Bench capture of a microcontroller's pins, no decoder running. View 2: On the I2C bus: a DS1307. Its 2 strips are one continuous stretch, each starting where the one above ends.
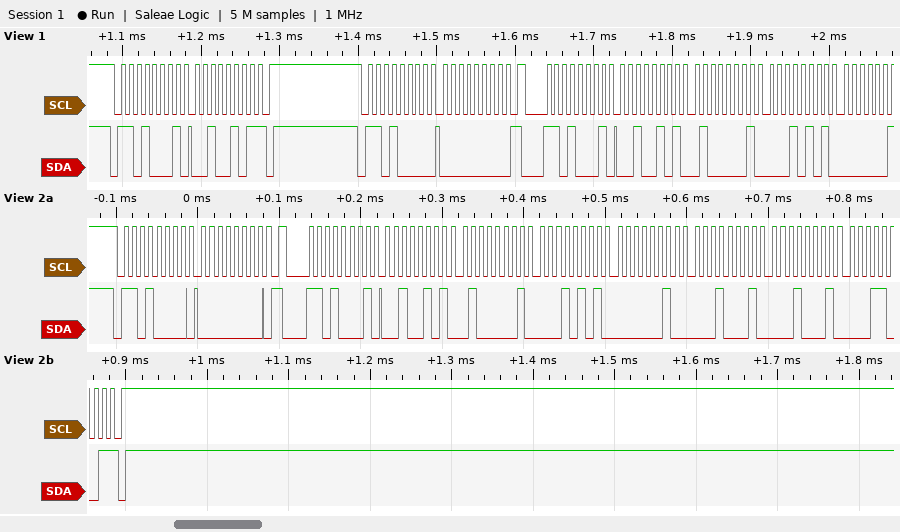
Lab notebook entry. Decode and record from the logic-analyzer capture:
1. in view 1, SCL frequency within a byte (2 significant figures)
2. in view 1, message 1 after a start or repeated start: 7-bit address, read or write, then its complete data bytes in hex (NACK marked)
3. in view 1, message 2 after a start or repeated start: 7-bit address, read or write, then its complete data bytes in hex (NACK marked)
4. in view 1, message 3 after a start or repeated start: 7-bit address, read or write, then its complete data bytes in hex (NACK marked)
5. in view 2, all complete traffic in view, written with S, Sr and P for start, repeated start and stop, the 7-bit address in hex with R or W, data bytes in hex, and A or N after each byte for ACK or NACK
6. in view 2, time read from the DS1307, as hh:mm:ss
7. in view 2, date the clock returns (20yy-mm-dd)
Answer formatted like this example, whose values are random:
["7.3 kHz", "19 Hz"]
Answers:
["100 kHz", "0x68 read: 25 NACK", "0x68 write: 00", "0x68 read: 25 41 15", "S 68W A 00 A Sr 68R A 25 A 41 A 15 A 02 A 11 A 11 A 19 N P", "15:41:25", "2019-11-11"]
